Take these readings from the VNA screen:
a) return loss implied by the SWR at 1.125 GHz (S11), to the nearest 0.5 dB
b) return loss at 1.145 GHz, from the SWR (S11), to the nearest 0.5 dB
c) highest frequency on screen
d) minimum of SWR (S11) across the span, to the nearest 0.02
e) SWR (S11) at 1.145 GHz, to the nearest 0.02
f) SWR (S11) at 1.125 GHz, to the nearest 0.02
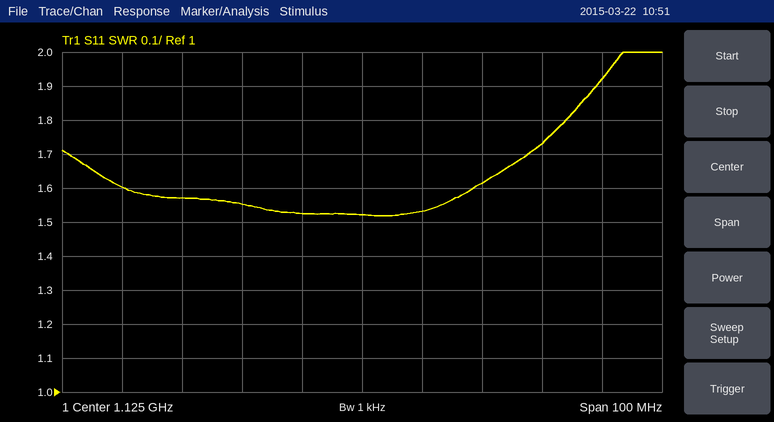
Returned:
13.5 dB
12.5 dB
1.175 GHz
1.52
1.62
1.52
